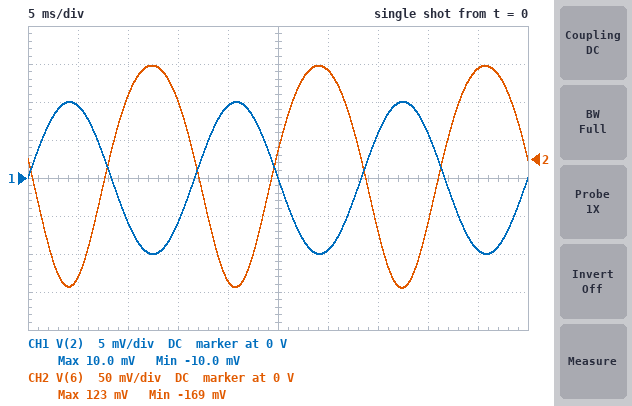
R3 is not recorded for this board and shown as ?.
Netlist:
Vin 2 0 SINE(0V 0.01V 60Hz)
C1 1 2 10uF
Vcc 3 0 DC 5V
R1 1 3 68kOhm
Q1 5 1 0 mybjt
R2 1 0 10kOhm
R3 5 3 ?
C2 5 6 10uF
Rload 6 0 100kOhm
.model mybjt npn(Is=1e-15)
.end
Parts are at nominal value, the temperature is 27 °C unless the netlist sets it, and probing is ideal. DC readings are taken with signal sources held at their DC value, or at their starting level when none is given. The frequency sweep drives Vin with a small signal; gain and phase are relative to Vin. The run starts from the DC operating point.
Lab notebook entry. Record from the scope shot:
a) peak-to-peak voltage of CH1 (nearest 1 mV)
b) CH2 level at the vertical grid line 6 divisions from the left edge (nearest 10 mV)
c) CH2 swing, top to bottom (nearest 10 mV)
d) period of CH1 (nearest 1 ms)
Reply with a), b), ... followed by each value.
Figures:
a) 20 mV
b) 120 mV
c) 290 mV
d) 17 ms
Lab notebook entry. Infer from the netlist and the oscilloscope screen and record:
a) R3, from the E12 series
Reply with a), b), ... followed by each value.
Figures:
a) 8.2 kΩ
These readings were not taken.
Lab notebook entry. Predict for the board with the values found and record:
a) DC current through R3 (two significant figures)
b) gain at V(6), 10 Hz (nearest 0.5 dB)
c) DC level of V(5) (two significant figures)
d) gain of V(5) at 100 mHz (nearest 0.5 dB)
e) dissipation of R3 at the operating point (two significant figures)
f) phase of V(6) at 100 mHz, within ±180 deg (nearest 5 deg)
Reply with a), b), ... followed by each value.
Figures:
a) 49 µA
b) 23.0 dB
c) 4.6 V
d) -3.0 dB
e) 20 µW
f) -35 deg
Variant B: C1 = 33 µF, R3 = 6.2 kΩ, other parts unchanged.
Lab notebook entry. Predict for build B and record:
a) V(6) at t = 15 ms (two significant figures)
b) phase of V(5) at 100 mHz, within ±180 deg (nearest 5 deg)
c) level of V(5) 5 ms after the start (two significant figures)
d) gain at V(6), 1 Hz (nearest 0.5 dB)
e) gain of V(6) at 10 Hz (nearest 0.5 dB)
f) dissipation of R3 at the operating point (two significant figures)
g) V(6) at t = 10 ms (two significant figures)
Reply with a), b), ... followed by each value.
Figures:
a) 59 mV
b) -100 deg
c) 4.6 V
d) 19.5 dB
e) 21.0 dB
f) 15 µW
g) 61 mV
